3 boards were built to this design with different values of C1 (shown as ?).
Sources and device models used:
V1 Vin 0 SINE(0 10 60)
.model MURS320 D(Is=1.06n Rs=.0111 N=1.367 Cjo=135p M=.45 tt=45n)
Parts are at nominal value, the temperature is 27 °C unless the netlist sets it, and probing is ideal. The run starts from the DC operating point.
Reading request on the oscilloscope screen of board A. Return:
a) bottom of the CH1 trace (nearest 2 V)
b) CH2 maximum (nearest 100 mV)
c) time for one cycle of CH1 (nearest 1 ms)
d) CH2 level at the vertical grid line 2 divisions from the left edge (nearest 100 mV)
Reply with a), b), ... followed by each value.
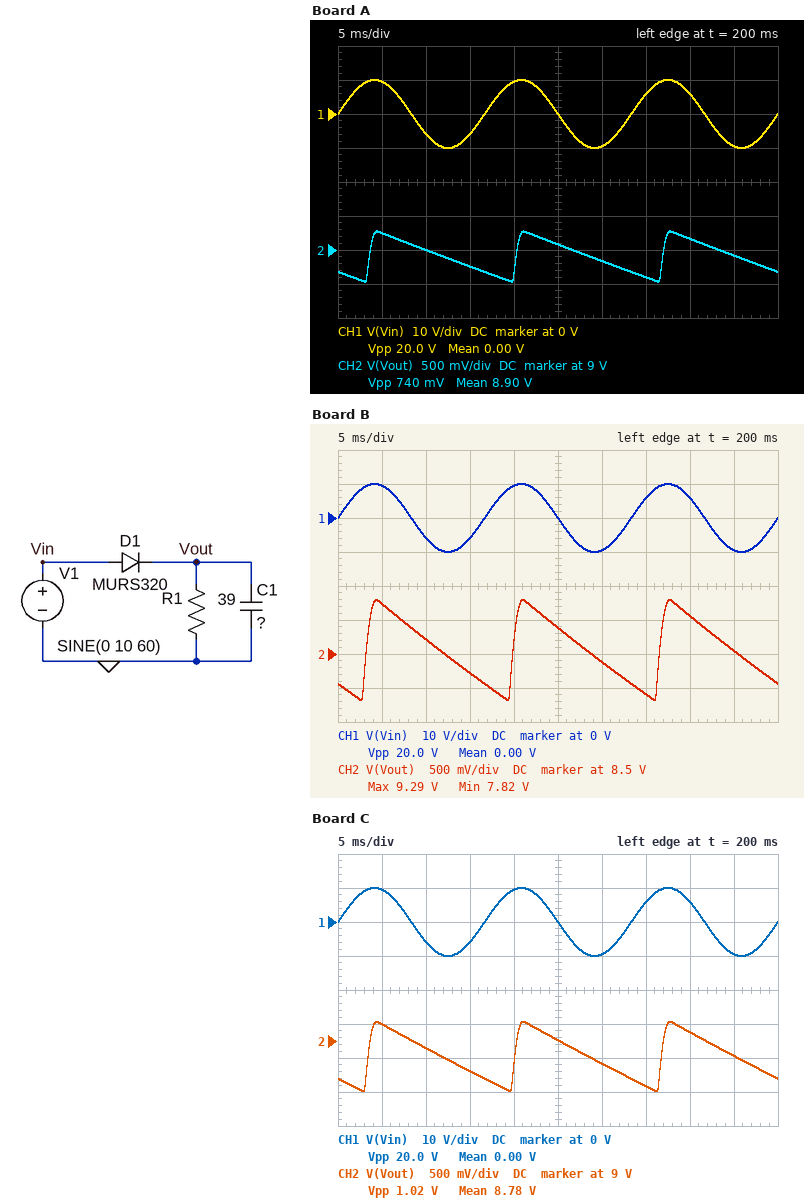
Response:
a) -10 V
b) 9.3 V
c) 17 ms
d) 9.0 V
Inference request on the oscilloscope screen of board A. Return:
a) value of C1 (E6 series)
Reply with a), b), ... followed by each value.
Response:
a) 4.7 mF
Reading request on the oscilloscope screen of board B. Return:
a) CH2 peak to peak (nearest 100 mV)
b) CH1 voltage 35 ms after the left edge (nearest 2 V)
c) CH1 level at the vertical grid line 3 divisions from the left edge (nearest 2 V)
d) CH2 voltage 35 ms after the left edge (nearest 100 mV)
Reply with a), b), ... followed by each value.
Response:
a) 1.5 V
b) 6 V
c) -6 V
d) 7.9 V
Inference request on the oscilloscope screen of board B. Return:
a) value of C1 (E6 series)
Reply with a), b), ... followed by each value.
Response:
a) 2.2 mF
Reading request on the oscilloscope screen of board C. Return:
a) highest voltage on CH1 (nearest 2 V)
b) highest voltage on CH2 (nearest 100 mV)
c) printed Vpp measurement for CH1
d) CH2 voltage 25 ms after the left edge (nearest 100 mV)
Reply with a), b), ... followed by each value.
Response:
a) 10 V
b) 9.3 V
c) 20.0 V
d) 9.0 V
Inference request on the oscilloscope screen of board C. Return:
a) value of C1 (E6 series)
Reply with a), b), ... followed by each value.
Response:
a) 3.3 mF
